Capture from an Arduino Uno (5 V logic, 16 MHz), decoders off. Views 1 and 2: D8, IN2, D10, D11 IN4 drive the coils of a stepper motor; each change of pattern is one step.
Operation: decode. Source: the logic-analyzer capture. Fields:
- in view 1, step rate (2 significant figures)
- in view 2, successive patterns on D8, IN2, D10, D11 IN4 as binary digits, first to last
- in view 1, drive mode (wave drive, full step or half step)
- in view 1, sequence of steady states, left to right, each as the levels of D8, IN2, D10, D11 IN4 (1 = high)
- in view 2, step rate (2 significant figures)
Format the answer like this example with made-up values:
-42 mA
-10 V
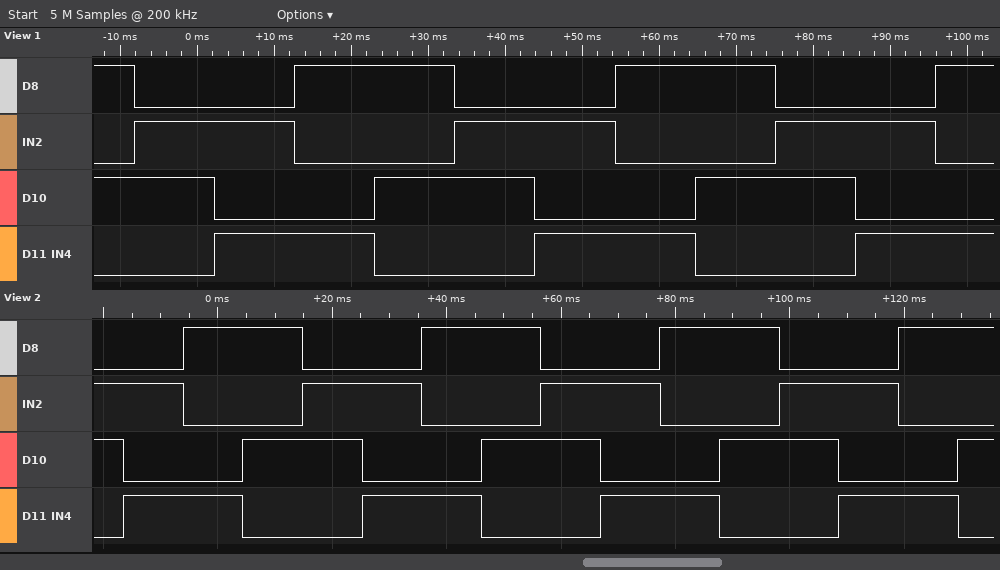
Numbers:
96 steps/s
0110 0101 1001 1010 0110 0101 1001 1010 0110 0101 1001 1010 0110 0101 1001 1010
full step
1010 0110 0101 1001 1010 0110 0101 1001 1010 0110 0101 1001
96 steps/s
